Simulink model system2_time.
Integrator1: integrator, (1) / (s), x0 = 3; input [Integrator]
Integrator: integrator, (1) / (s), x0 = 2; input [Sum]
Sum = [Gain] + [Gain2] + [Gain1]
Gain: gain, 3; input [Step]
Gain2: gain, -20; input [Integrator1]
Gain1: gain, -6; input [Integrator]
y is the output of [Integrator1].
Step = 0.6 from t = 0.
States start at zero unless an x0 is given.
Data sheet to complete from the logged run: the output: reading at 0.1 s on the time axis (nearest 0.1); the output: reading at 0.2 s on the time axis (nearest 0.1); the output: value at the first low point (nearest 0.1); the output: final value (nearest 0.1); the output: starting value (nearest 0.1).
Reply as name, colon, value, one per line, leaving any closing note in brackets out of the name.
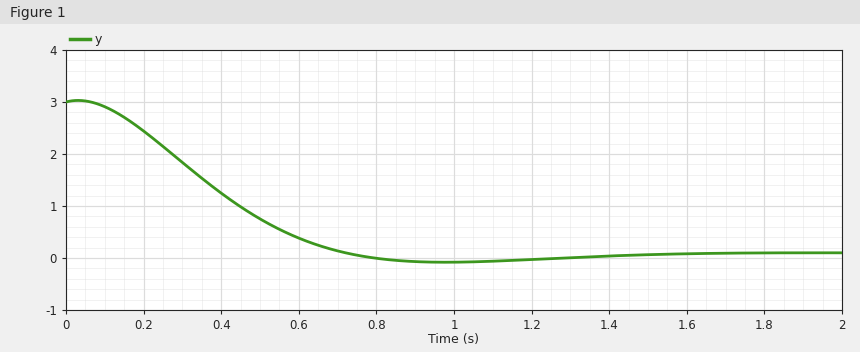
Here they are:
the output: reading at 0.1 s on the time axis: 2.9
the output: reading at 0.2 s on the time axis: 2.4
the output: value at the first low point: -0.1
the output: final value: 0.1
the output: starting value: 3.0
